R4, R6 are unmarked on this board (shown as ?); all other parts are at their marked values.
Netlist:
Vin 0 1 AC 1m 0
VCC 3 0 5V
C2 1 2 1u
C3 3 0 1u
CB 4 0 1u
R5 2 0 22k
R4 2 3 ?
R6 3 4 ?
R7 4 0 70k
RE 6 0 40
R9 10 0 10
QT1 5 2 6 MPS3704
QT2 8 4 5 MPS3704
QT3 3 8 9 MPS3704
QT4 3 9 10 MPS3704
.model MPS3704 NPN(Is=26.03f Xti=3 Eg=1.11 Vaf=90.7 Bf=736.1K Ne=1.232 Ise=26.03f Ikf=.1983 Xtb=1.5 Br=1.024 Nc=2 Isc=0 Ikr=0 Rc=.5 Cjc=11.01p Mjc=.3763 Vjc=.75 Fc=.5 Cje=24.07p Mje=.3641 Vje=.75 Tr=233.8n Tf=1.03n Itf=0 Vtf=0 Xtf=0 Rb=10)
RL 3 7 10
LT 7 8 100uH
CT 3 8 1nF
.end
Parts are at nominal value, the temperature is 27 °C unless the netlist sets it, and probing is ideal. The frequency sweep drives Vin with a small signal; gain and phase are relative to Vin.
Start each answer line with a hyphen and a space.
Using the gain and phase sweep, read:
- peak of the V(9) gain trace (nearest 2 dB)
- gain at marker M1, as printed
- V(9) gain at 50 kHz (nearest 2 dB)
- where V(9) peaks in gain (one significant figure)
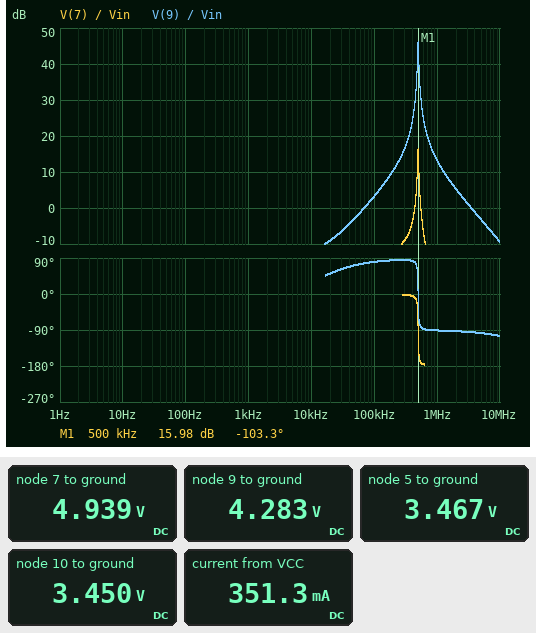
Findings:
- 46 dB
- 15.98 dB
- -2 dB
- 500 kHz
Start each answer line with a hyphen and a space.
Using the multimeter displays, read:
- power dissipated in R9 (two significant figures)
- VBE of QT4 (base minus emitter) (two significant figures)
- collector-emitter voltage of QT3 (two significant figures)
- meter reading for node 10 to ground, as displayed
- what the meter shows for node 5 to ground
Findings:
- 1.2 W
- 830 mV
- 720 mV
- 3.450 V
- 3.467 V
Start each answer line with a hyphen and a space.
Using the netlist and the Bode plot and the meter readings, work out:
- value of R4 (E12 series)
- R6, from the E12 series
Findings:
- 47 kΩ
- 8.2 kΩ
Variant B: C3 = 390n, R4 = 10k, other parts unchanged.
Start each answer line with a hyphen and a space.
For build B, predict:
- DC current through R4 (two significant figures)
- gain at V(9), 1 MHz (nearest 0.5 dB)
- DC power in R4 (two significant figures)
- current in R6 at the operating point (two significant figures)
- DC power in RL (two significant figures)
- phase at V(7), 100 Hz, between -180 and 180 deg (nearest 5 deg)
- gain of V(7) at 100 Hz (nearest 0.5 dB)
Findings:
- 290 µA
- 14.0 dB
- 860 µW
- 240 µA
- 11 mW
- 25 deg
- -13.0 dB
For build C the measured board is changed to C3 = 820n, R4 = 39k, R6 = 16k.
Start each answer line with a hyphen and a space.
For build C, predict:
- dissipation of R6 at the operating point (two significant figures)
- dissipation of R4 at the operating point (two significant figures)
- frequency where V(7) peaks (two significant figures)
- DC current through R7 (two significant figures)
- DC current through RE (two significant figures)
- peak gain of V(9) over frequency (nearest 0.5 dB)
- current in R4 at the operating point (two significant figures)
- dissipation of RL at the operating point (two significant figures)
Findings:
- 170 µW
- 410 µW
- 500 kHz
- 48 µA
- 8.1 mA
- 46.5 dB
- 100 µA
- 650 µW
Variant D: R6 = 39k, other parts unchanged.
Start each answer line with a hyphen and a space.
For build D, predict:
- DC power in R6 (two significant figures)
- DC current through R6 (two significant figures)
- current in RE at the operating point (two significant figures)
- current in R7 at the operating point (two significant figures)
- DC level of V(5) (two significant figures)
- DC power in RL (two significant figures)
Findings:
- 210 µW
- 74 µA
- 6.1 mA
- 30 µA
- 1.4 V
- 370 µW
